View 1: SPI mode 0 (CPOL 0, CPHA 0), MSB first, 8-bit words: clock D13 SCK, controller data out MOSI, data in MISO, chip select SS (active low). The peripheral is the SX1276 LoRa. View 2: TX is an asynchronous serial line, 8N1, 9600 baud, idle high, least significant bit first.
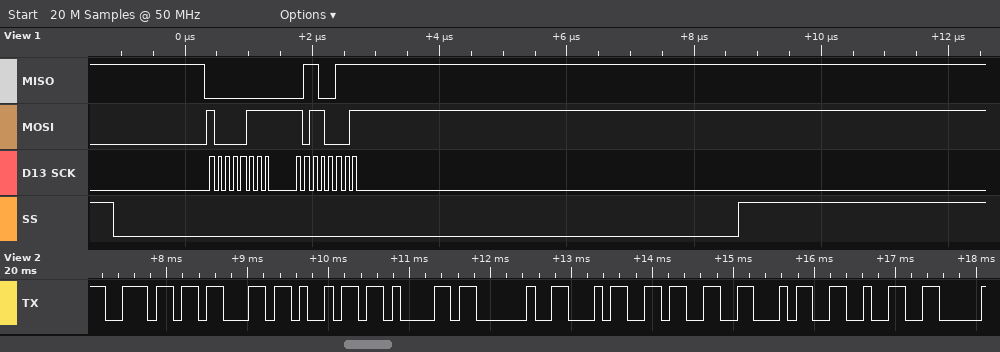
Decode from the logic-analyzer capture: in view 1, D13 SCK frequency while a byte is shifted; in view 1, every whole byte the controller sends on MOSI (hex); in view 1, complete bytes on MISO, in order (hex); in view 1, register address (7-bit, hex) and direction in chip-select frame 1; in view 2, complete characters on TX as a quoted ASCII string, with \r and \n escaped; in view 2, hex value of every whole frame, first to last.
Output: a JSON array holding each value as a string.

["8 MHz", "87 B1", "00 67", "0x07 write", "\"ncia 4342\"", "0x6E 0x63 0x69 0x61 0x20 0x34 0x33 0x34 0x32"]
